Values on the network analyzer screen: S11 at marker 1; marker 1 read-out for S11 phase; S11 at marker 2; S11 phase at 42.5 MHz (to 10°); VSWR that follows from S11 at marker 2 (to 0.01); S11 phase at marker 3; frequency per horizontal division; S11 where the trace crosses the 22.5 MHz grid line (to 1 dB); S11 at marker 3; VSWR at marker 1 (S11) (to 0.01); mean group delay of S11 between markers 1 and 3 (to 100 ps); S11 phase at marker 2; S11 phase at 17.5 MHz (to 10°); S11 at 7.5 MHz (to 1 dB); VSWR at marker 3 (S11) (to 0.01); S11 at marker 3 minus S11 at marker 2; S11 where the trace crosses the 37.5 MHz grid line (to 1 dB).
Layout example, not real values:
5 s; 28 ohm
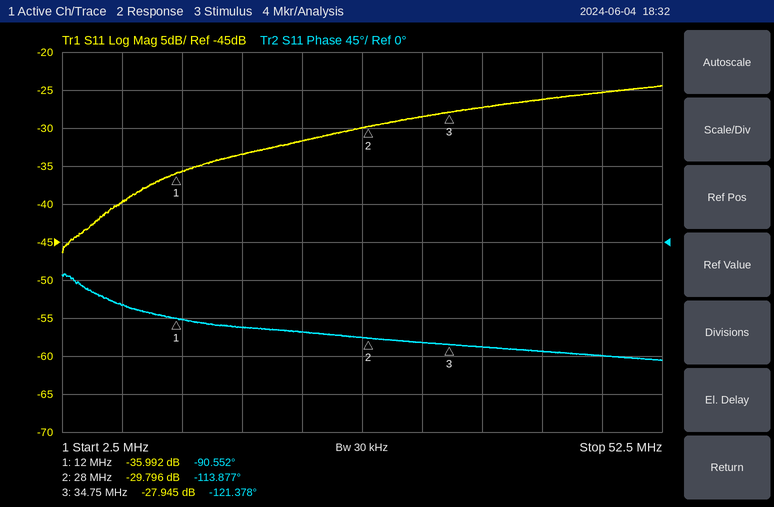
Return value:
-35.992 dB; -90.552°; -29.796 dB; -130°; 1.07; -121.378°; 5 MHz; -32 dB; -27.945 dB; 1.03; 3.8 ns; -113.877°; -100°; -40 dB; 1.08; 1.851 dB; -27 dB
